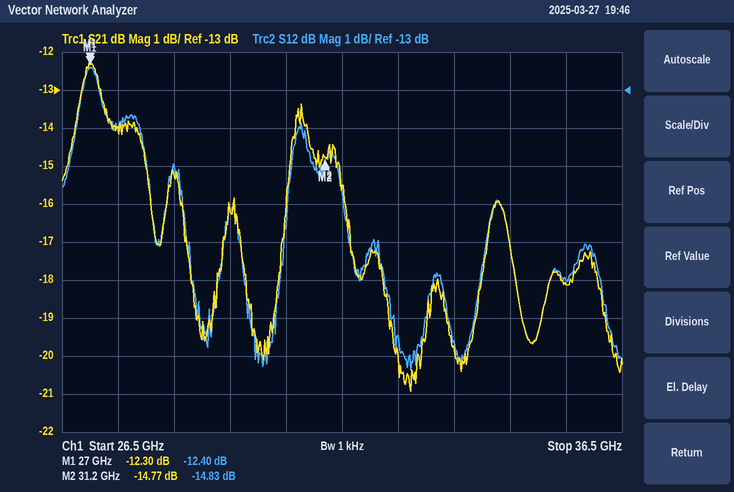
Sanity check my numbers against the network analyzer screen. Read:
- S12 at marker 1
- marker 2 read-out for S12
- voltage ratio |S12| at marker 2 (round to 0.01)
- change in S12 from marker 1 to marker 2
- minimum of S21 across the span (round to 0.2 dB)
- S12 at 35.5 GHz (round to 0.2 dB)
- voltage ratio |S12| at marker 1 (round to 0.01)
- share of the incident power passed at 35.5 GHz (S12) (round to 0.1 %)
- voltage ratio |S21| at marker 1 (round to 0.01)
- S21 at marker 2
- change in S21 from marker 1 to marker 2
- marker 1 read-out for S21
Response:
-12.40 dB
-14.83 dB
0.18
-2.43 dB
-21.0 dB
-18.0 dB
0.24
1.6 %
0.24
-14.77 dB
-2.47 dB
-12.30 dB
